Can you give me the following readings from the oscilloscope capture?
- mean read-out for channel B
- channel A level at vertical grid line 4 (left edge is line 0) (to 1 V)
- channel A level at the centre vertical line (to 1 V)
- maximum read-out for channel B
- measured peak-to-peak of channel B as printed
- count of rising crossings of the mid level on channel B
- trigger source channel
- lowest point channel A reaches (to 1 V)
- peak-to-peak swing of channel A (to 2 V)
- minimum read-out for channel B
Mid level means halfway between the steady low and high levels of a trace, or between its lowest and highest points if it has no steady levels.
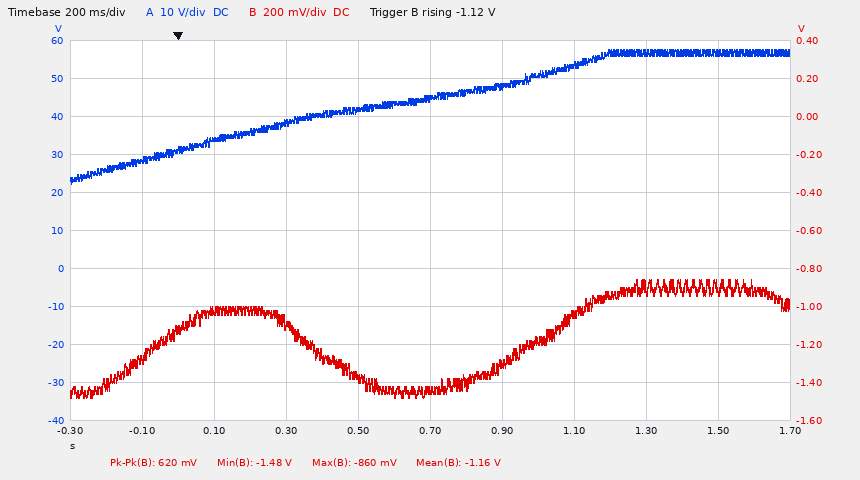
-1.16 V
42 V
45 V
-860 mV
620 mV
2
channel B
22 V
36 V
-1.48 V
